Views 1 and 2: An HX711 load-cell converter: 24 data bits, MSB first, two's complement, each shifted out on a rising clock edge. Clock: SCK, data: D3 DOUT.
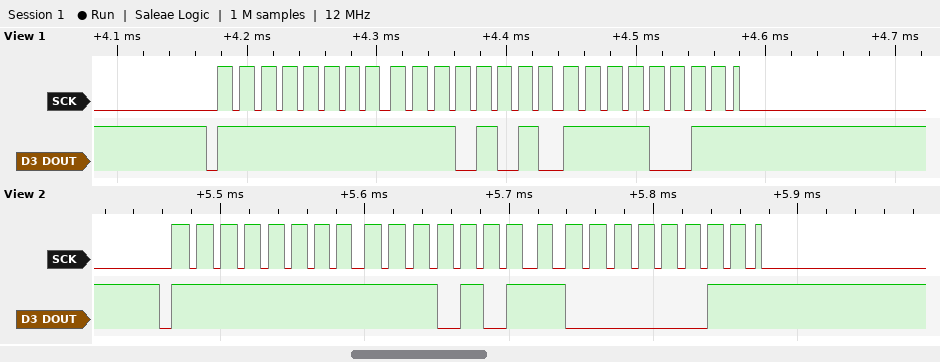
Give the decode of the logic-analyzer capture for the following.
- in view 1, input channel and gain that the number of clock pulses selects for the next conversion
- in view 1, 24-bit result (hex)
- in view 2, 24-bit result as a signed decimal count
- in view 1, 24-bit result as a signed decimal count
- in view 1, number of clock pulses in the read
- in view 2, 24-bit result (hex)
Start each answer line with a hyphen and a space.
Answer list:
- channel A, gain 128
- 0xFFEAF3
- -5373
- -5389
- 25
- 0xFFEB03
